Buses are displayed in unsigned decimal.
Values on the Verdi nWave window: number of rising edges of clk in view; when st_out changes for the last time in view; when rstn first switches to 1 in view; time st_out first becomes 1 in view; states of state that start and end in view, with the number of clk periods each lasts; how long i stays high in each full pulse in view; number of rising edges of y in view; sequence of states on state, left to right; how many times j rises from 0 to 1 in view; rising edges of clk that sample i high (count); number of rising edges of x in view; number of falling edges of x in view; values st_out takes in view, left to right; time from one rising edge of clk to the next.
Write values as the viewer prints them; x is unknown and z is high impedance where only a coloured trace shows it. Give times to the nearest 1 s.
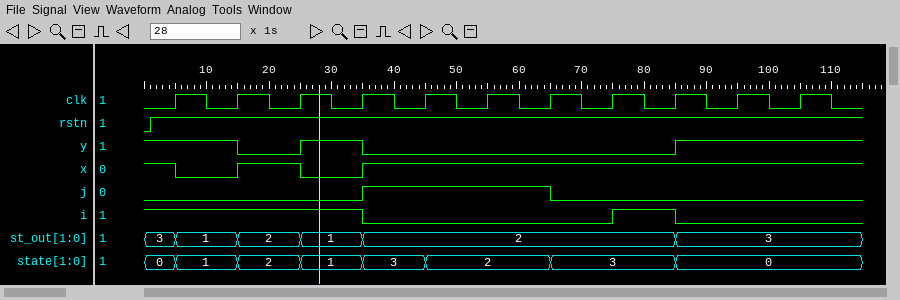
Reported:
11
85 s
1 s
5 s
1: 1, 2: 1, 1: 1, 3: 1, 2: 2, 3: 2
10 s
2
0, 1, 2, 1, 3, 2, 3, 0
1
5
2
2
3, 1, 2, 1, 2, 3
10 s
